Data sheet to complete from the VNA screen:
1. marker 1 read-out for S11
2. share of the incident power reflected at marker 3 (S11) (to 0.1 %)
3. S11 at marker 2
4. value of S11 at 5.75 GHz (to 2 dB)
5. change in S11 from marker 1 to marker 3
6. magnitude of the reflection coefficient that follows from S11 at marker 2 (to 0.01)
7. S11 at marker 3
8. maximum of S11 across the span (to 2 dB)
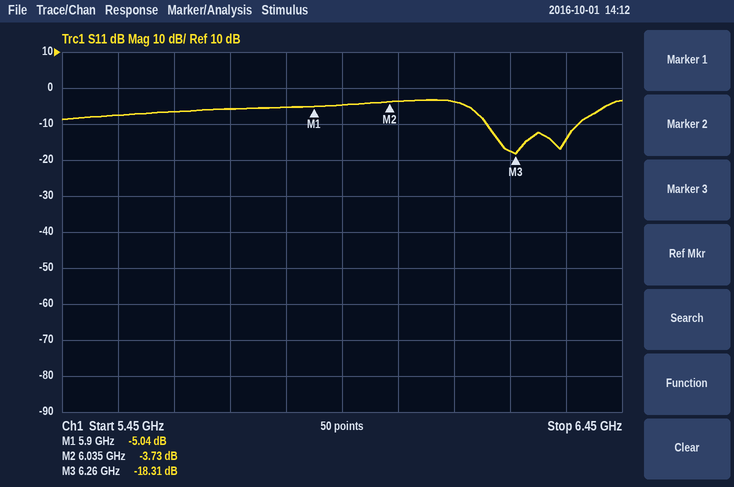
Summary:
-5.04 dB
1.5 %
-3.73 dB
-6 dB
-13.27 dB
0.65
-18.31 dB
-4 dB
